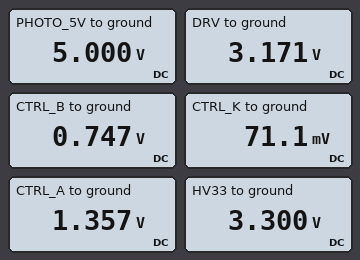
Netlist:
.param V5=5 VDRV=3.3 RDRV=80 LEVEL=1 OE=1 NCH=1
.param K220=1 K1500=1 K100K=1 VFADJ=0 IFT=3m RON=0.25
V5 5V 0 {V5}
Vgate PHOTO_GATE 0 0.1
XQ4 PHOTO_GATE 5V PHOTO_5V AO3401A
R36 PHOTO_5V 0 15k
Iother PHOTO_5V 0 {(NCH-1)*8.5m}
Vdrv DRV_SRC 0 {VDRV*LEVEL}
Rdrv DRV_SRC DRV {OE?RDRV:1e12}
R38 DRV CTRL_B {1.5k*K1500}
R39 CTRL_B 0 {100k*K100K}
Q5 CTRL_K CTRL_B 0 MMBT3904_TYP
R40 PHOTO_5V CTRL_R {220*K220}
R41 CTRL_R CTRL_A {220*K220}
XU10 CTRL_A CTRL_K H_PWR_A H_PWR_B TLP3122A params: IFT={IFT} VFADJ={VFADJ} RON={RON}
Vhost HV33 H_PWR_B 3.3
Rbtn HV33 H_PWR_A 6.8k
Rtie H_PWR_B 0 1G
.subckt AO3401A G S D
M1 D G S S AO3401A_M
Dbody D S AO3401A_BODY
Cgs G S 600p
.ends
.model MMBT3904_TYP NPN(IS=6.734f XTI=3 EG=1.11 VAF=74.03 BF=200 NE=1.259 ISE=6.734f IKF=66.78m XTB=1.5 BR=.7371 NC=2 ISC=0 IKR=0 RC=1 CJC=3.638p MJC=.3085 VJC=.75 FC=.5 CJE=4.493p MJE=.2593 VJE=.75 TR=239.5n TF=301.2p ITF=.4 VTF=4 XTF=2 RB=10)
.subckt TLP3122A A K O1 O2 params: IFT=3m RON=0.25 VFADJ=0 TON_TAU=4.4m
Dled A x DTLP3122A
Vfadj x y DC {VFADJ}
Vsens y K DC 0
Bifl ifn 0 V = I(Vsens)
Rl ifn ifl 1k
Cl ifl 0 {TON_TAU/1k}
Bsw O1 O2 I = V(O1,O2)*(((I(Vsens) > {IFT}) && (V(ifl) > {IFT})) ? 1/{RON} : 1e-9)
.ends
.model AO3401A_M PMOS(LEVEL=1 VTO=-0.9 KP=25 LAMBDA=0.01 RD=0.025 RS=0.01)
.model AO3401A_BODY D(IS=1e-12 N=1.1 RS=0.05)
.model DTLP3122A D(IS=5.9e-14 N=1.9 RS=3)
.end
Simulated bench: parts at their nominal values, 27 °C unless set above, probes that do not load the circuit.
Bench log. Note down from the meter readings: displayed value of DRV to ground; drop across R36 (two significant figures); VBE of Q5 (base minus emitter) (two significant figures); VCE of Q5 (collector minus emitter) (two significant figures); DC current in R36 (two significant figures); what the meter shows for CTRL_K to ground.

3.171 V
5.0 V
750 mV
71 mV
330 µA
71.1 mV
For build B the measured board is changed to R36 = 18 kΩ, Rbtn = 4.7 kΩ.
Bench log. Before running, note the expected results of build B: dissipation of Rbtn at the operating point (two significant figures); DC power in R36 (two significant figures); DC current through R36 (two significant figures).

2.3 mW
1.4 mW
280 µA
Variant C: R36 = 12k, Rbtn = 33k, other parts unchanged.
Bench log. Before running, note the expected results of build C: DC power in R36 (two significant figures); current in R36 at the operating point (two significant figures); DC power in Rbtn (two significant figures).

2.1 mW
420 µA
330 µW
